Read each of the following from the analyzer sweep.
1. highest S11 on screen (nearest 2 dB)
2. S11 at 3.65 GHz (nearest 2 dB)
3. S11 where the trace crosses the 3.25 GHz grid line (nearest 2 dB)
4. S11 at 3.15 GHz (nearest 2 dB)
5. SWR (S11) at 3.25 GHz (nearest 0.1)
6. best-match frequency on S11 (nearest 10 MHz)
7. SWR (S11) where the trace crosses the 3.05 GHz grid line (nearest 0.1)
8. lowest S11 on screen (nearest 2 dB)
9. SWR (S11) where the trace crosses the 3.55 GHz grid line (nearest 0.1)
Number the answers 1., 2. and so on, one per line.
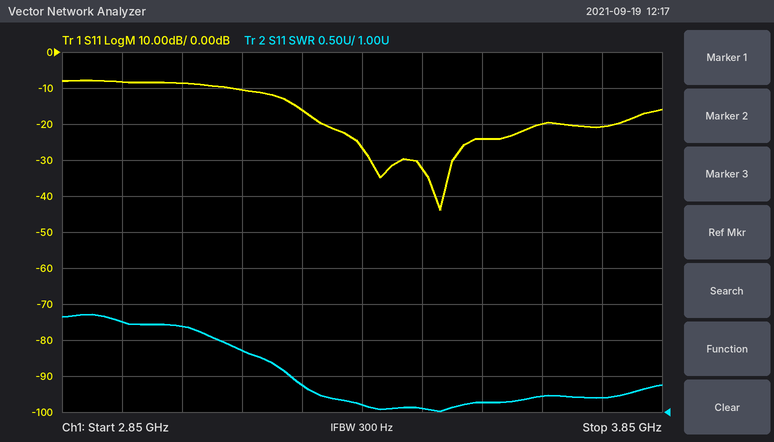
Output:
1. -8 dB
2. -20 dB
3. -16 dB
4. -10 dB
5. 1.4
6. 3.48 GHz
7. 2.2
8. -44 dB
9. 1.1
